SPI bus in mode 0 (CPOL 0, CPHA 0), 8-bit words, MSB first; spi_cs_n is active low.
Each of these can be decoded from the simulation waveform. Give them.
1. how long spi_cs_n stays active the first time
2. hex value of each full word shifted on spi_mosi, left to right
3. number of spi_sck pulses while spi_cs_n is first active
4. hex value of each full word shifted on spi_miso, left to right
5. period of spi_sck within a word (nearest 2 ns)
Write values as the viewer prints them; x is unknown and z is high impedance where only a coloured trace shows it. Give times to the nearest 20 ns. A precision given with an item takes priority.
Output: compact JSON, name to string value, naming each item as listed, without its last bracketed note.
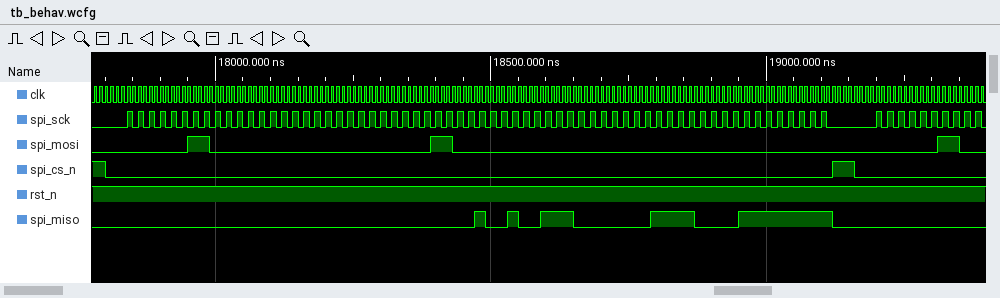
{"how long spi_cs_n stays active the first time": "1320 ns", "hex value of each full word shifted on spi_mosi, left to right": "03, 00, 00, 0C, 00, 00, 00, 00, 03", "number of spi_sck pulses while spi_cs_n is first active": "64", "hex value of each full word shifted on spi_miso, left to right": "00, 00, 00, 00, 93, 80, F0, FF, 00", "period of spi_sck within a word": "20 ns"}
